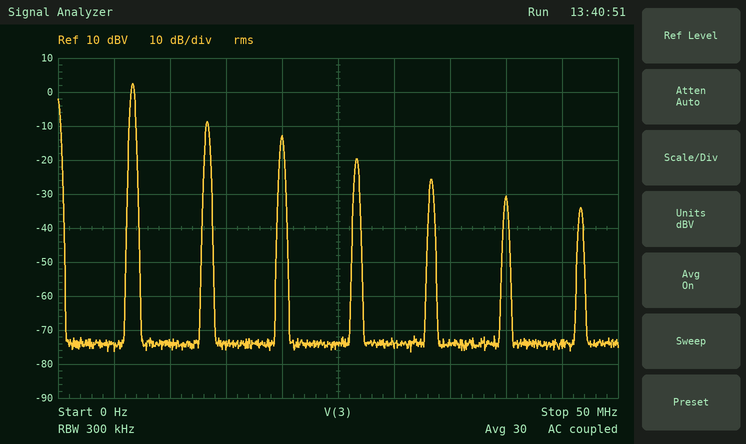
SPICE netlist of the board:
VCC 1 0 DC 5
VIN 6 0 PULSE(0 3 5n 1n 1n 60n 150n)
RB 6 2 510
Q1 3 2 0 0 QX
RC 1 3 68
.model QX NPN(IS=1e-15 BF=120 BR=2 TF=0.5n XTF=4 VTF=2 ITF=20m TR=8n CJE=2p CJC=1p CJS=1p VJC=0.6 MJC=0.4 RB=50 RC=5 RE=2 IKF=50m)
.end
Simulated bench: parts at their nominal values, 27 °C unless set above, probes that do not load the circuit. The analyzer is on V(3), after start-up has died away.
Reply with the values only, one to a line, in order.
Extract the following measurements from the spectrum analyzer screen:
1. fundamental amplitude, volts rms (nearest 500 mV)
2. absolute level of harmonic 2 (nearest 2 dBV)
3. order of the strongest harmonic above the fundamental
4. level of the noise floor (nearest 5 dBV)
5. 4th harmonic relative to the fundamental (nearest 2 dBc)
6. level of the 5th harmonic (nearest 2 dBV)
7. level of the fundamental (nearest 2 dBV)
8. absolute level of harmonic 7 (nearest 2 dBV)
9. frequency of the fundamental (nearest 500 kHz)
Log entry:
1.5 V
-8 dBV
2
-75 dBV
-22 dBc
-26 dBV
2 dBV
-34 dBV
6.5 MHz
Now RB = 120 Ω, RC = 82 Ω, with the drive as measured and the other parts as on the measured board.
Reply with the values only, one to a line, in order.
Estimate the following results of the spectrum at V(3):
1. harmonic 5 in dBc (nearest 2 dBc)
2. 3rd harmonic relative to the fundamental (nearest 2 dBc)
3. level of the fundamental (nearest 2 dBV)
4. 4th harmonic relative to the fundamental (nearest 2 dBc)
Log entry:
-24 dBc
-16 dBc
6 dBV
-14 dBc
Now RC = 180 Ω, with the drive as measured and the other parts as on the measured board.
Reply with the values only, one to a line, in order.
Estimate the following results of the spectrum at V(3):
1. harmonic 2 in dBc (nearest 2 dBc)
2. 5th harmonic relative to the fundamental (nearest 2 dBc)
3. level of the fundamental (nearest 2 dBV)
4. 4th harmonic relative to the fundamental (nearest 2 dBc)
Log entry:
-8 dBc
-20 dBc
6 dBV
-16 dBc
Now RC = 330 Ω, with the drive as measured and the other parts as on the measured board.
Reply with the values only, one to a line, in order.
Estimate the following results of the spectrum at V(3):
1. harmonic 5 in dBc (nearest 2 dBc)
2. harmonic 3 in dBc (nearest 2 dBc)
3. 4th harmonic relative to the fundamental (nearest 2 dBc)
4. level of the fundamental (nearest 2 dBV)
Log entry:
-32 dBc
-14 dBc
-14 dBc
6 dBV
